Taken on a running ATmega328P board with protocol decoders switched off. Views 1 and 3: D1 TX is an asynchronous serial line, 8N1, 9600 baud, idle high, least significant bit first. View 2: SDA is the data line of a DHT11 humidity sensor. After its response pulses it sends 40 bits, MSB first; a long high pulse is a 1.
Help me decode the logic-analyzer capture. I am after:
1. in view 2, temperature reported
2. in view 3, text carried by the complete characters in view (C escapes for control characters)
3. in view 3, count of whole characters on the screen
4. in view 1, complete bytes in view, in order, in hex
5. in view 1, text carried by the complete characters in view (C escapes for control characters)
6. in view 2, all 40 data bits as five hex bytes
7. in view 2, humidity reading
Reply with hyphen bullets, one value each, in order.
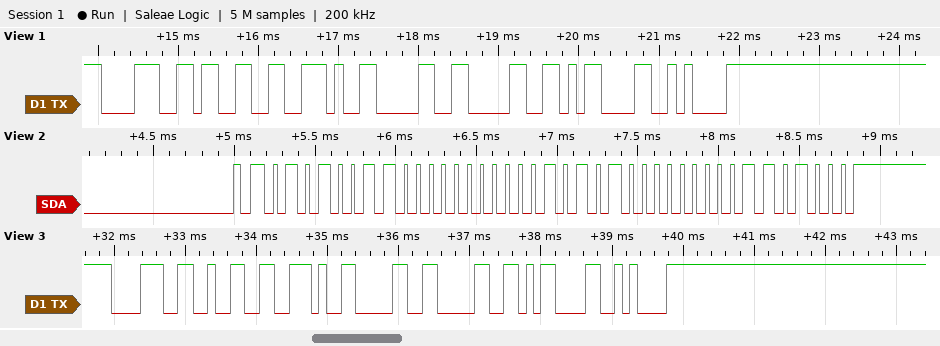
- 21.0 °C
- "82.00\r\n"
- 7
- 38 33 2E 30 30 0D 0A
- "83.00\r\n"
- 53 00 15 00 68
- 83 %
